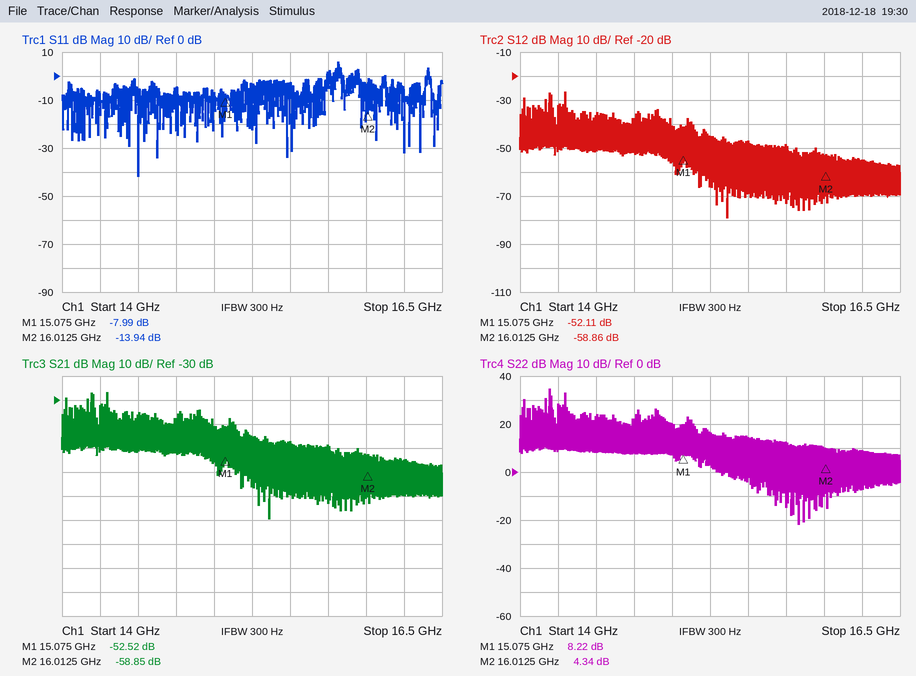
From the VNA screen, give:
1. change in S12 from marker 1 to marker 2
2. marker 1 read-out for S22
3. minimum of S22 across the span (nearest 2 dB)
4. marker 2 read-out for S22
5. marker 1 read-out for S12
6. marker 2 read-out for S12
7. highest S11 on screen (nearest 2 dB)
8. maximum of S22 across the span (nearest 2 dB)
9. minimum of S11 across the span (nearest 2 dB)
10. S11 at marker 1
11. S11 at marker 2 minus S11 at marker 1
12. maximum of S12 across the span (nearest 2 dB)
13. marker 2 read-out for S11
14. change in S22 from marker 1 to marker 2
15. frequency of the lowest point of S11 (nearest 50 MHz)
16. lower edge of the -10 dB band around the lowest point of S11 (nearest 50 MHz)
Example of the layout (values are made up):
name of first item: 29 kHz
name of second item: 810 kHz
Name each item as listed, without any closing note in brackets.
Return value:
change in S12 from marker 1 to marker 2: -6.75 dB
marker 1 read-out for S22: 8.22 dB
minimum of S22 across the span: -22 dB
marker 2 read-out for S22: 4.34 dB
marker 1 read-out for S12: -52.11 dB
marker 2 read-out for S12: -58.86 dB
highest S11 on screen: 6 dB
maximum of S22 across the span: 34 dB
minimum of S11 across the span: -42 dB
S11 at marker 1: -7.99 dB
S11 at marker 2 minus S11 at marker 1: -5.95 dB
maximum of S12 across the span: -26 dB
marker 2 read-out for S11: -13.94 dB
change in S22 from marker 1 to marker 2: -3.88 dB
frequency of the lowest point of S11: 14.50 GHz
lower edge of the -10 dB band around the lowest point of S11: 14.50 GHz
